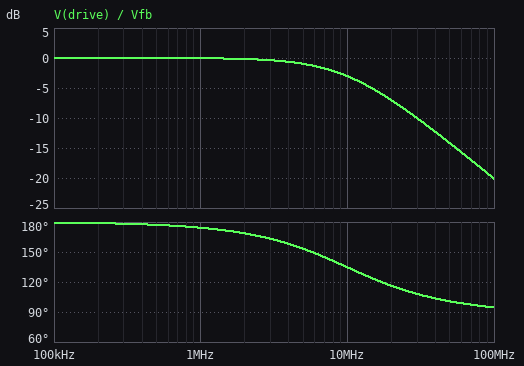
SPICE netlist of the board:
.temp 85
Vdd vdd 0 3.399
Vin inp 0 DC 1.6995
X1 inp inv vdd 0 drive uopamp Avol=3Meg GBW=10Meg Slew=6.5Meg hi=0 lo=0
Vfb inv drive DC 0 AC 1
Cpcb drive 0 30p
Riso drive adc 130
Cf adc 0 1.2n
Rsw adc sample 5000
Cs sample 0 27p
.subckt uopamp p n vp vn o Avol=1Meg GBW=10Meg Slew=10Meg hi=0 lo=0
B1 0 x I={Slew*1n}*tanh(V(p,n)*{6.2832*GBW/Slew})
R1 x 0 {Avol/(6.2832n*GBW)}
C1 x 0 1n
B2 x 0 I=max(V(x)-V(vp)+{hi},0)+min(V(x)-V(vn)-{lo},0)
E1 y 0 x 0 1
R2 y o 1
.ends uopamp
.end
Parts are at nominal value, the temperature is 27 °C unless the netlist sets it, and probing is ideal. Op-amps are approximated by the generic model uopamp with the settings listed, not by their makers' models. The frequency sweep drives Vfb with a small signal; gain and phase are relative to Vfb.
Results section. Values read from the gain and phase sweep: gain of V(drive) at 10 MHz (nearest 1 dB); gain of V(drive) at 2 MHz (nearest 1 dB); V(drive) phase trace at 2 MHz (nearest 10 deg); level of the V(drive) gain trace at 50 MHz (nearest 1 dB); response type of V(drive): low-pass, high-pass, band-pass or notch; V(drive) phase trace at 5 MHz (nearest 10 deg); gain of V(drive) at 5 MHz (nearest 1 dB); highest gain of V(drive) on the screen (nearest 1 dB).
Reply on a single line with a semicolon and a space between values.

-3 dB; 0 dB; 170 deg; -14 dB; low-pass; 150 deg; -1 dB; 0 dB
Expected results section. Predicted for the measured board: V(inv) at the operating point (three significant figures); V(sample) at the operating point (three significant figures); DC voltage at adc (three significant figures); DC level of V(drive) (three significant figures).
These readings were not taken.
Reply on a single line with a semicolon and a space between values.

1.70 V; 1.70 V; 1.70 V; 1.70 V
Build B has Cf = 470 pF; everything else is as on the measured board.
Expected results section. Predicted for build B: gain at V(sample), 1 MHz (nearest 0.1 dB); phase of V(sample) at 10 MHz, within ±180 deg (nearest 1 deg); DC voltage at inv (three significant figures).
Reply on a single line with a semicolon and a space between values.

-3.1 dB; -24 deg; 1.70 V
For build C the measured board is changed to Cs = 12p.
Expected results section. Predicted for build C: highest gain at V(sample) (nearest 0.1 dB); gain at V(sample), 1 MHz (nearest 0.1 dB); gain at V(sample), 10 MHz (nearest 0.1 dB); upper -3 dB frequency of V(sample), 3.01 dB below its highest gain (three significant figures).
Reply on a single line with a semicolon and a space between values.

0 dB; -3.6 dB; -34.7 dB; 892 kHz
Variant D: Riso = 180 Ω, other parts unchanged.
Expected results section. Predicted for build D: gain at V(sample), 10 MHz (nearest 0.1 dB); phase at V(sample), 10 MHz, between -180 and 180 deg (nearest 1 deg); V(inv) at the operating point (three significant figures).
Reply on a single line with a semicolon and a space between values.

-44.3 dB; -34 deg; 1.70 V
